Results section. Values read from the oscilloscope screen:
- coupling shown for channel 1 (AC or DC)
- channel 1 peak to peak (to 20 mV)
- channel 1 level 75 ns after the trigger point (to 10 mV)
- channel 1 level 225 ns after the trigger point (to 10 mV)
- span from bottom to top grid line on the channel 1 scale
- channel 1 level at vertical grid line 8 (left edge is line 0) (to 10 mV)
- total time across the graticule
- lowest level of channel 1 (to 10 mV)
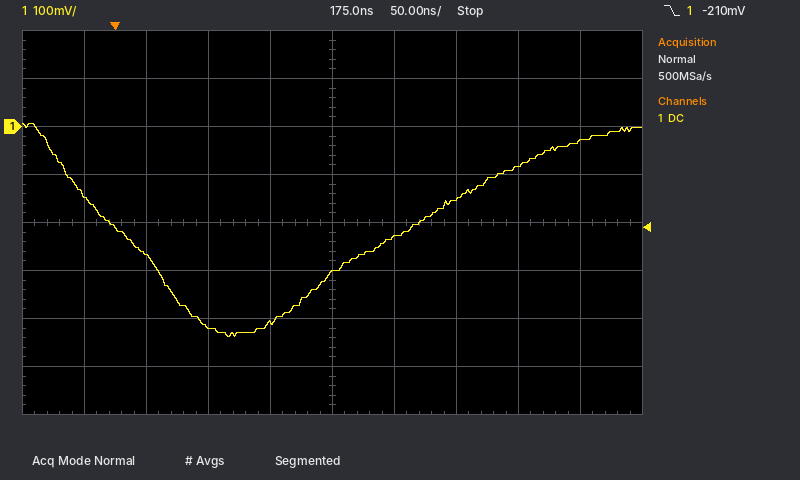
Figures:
DC
440 mV
-420 mV
-230 mV
800 mV
-80 mV
500 ns
-440 mV
